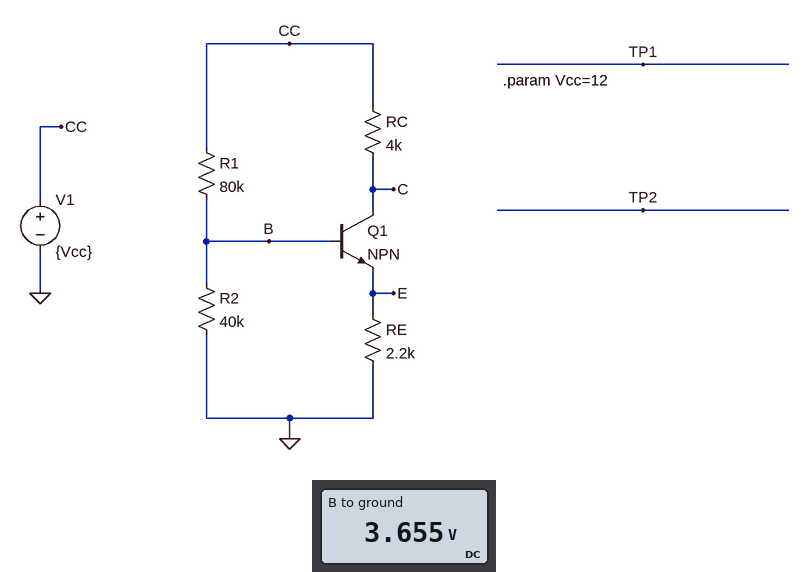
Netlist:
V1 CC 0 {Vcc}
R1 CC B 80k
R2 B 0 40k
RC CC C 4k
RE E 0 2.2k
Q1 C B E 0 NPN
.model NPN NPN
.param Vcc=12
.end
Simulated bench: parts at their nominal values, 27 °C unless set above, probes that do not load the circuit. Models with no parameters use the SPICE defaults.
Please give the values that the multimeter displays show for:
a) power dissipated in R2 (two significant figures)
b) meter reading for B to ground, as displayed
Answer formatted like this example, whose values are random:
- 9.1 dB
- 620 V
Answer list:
- 330 µW
- 3.655 V
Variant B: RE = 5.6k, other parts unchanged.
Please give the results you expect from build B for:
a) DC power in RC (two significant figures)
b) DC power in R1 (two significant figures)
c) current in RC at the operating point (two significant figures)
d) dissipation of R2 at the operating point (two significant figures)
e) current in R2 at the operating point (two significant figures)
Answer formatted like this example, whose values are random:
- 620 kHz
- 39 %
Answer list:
- 1.2 mW
- 830 µW
- 550 µA
- 370 µW
- 96 µA
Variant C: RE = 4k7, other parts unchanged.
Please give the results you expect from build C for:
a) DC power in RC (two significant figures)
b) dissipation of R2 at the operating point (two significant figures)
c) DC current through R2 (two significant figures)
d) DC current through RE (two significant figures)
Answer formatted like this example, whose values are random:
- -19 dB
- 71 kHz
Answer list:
- 1.7 mW
- 370 µW
- 96 µA
- 650 µA
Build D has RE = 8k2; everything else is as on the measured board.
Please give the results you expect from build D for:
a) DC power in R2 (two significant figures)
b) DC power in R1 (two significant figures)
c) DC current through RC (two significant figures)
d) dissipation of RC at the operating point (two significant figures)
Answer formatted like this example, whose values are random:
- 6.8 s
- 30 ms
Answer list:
- 380 µW
- 820 µW
- 380 µA
- 580 µW
